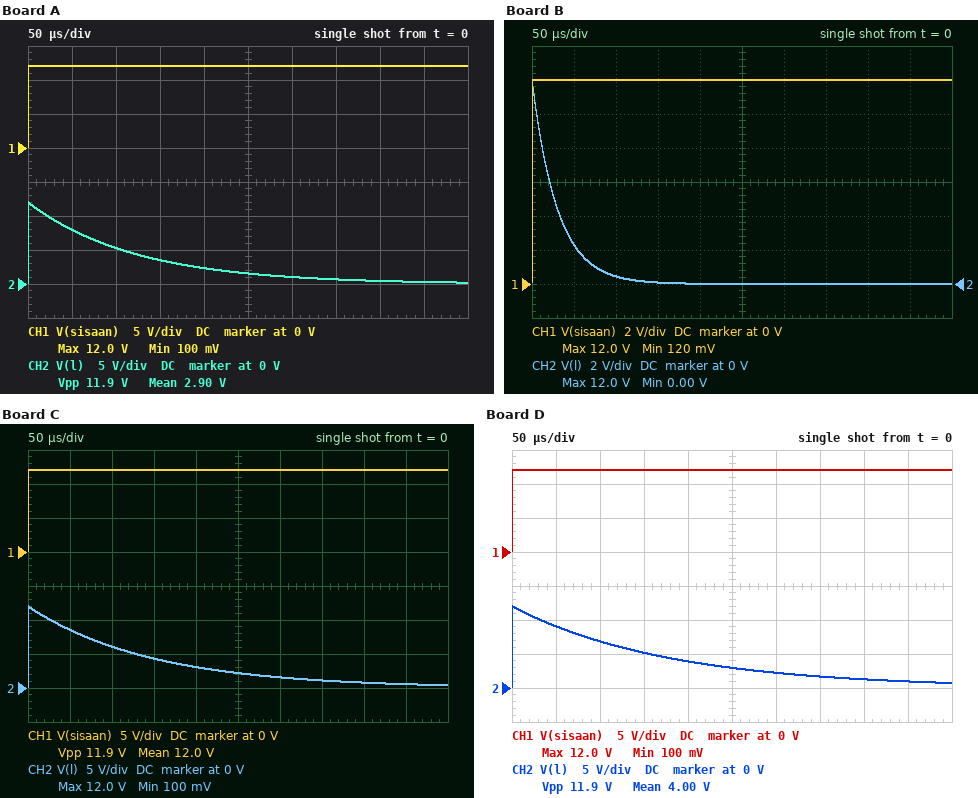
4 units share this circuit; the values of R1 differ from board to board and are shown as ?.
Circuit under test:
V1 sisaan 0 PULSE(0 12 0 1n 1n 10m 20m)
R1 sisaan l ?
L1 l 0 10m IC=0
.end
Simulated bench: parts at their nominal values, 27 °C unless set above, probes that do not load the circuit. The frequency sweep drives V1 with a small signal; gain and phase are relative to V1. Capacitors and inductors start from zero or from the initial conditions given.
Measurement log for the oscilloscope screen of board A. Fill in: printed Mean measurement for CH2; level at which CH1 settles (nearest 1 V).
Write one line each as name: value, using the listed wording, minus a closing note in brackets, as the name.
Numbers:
printed Mean measurement for CH2: 2.90 V
level at which CH1 settles: 12 V
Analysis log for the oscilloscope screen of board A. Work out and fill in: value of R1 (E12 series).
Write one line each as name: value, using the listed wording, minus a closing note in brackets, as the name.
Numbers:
value of R1: 82 Ω
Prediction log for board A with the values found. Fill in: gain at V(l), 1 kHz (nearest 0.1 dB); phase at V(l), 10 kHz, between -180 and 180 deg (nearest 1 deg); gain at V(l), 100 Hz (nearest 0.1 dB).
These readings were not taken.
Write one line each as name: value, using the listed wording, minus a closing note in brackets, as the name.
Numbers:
gain at V(l), 1 kHz: -4.3 dB
phase at V(l), 10 kHz, between -180 and 180 deg: 7 deg
gain at V(l), 100 Hz: -22.3 dB
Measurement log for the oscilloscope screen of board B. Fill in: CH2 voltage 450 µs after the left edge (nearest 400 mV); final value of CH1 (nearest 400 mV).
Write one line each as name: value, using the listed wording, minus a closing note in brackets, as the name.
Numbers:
CH2 voltage 450 µs after the left edge: 0 V
final value of CH1: 12.0 V
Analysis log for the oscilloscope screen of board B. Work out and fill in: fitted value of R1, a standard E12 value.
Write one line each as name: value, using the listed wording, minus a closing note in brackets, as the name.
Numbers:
fitted value of R1, a standard E12 value: 330 Ω
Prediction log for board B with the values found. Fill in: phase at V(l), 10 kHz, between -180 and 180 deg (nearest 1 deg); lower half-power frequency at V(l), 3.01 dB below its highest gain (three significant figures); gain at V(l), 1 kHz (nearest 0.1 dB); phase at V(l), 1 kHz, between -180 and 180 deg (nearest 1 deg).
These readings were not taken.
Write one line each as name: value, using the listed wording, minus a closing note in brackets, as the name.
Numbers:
phase at V(l), 10 kHz, between -180 and 180 deg: 28 deg
lower half-power frequency at V(l), 3.01 dB below its highest gain: 5.25 kHz
gain at V(l), 1 kHz: -14.6 dB
phase at V(l), 1 kHz, between -180 and 180 deg: 79 deg
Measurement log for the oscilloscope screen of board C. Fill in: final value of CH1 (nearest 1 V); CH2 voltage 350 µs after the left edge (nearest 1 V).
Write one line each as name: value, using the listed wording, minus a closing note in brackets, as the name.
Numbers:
final value of CH1: 12 V
CH2 voltage 350 µs after the left edge: 1 V
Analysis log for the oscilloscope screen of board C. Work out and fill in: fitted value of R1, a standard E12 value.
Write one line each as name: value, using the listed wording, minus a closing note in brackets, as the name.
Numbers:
fitted value of R1, a standard E12 value: 68 Ω
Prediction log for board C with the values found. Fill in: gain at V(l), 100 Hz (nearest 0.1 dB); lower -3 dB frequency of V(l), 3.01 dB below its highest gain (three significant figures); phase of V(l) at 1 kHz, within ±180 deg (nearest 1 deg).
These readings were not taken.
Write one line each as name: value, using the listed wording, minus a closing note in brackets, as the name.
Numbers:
gain at V(l), 100 Hz: -20.7 dB
lower -3 dB frequency of V(l), 3.01 dB below its highest gain: 1.08 kHz
phase of V(l) at 1 kHz, within ±180 deg: 47 deg
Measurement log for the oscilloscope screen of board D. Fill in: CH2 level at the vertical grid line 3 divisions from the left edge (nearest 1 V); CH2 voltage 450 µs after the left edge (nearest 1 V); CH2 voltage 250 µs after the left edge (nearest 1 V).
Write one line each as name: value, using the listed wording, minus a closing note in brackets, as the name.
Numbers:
CH2 level at the vertical grid line 3 divisions from the left edge: 5 V
CH2 voltage 450 µs after the left edge: 1 V
CH2 voltage 250 µs after the left edge: 3 V
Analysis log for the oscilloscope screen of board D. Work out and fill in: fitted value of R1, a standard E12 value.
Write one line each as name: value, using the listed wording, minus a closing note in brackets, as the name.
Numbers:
fitted value of R1, a standard E12 value: 56 Ω
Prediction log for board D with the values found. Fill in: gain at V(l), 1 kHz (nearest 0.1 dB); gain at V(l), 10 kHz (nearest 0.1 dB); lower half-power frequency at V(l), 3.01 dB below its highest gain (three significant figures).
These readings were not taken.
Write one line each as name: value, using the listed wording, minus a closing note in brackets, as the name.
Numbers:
gain at V(l), 1 kHz: -2.5 dB
gain at V(l), 10 kHz: 0 dB
lower half-power frequency at V(l), 3.01 dB below its highest gain: 891 Hz
